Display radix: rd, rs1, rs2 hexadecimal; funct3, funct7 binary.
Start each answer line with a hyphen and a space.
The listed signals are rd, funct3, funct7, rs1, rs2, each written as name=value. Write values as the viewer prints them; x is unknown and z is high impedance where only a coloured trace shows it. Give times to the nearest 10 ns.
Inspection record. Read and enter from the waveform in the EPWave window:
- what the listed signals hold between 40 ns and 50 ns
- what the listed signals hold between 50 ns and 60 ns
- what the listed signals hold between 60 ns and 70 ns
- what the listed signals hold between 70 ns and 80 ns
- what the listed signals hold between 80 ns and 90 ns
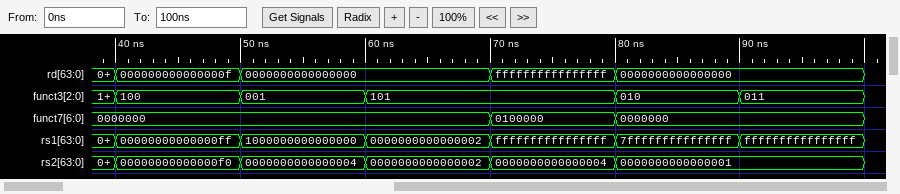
- rd=000000000000000f, funct3=100, funct7=0000000, rs1=00000000000000ff, rs2=00000000000000f0
- rd=0000000000000000, funct3=001, funct7=0000000, rs1=1000000000000000, rs2=0000000000000004
- rd=0000000000000000, funct3=101, funct7=0000000, rs1=0000000000000002, rs2=0000000000000002
- rd=ffffffffffffffff, funct3=101, funct7=0100000, rs1=ffffffffffffffff, rs2=0000000000000004
- rd=0000000000000000, funct3=010, funct7=0000000, rs1=7fffffffffffffff, rs2=0000000000000001
